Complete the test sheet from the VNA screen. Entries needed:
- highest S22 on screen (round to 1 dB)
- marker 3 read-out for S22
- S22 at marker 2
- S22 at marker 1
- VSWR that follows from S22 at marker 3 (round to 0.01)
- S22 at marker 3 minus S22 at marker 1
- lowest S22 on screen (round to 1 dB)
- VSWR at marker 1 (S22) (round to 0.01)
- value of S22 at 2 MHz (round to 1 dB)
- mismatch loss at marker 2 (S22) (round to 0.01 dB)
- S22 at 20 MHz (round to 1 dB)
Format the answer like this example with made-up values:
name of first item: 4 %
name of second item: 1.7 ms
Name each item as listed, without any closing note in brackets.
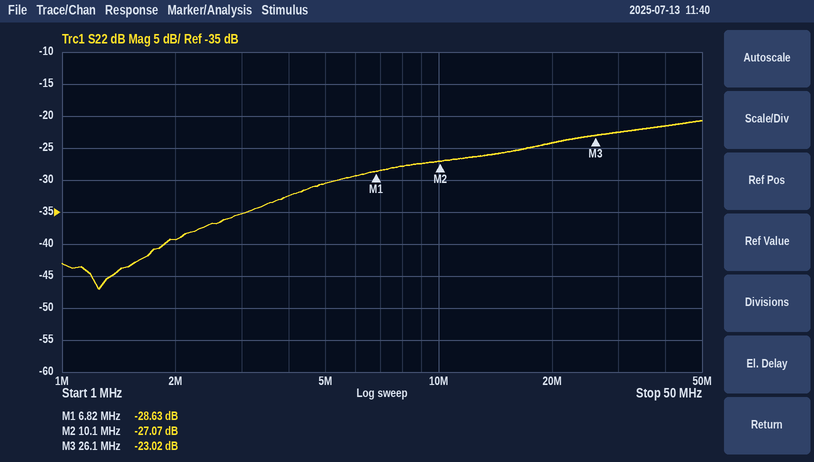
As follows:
highest S22 on screen: -21 dB
marker 3 read-out for S22: -23.02 dB
S22 at marker 2: -27.07 dB
S22 at marker 1: -28.63 dB
VSWR that follows from S22 at marker 3: 1.15
S22 at marker 3 minus S22 at marker 1: 5.61 dB
lowest S22 on screen: -47 dB
VSWR at marker 1 (S22): 1.08
value of S22 at 2 MHz: -39 dB
mismatch loss at marker 2 (S22): 0.01 dB
S22 at 20 MHz: -24 dB
